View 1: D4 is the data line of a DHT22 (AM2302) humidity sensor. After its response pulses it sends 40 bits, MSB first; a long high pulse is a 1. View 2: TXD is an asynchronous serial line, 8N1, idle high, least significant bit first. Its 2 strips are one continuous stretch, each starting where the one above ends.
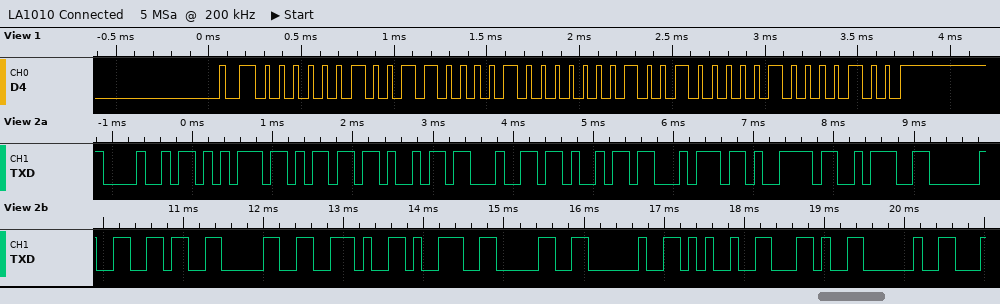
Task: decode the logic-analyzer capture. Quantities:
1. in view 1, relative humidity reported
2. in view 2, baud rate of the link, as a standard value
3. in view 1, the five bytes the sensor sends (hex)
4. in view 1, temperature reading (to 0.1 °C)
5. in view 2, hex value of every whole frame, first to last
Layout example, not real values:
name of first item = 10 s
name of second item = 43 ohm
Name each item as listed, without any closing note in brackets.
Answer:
in view 1, relative humidity reported = 60.9 %
in view 2, baud rate of the link, as a standard value = 9600 baud
in view 1, the five bytes the sensor sends = 02 61 01 20 84
in view 1, temperature reading = 28.8 °C
in view 2, hex value of every whole frame, first to last = 48 75 6D 69 64 69 74 79 3A 20 36 30 2E 39 30 20 25 2C 20
